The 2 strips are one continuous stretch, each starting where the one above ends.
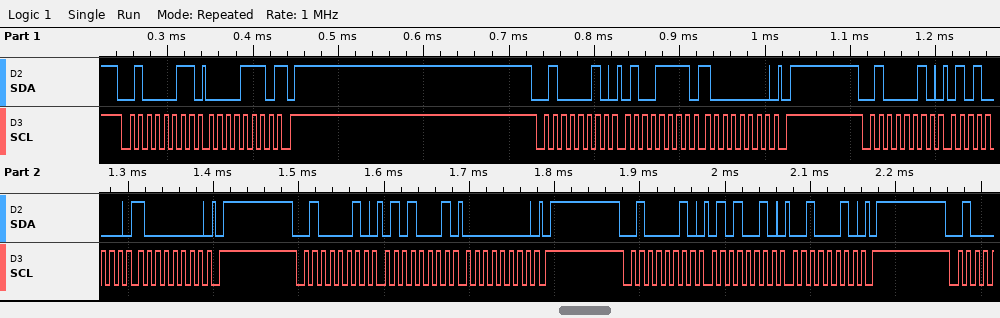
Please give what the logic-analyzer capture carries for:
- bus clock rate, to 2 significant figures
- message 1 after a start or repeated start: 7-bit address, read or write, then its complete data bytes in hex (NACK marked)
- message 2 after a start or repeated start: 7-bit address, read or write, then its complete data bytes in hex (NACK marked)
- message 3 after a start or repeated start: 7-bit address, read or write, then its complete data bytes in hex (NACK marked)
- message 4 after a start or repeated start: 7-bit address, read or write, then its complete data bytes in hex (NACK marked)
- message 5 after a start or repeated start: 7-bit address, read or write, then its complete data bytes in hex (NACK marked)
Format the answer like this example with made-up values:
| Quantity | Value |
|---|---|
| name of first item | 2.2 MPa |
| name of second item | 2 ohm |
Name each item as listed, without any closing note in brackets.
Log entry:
| Quantity | Value |
|---|---|
| bus clock rate, to 2 significant figures | 100 kHz |
| message 1 after a start or repeated start: 7-bit address, read or write, then its complete data bytes in hex | 0x21 read: 0E NACK |
| message 2 after a start or repeated start: 7-bit address, read or write, then its complete data bytes in hex | 0x21 write: 4F 80 |
| message 3 after a start or repeated start: 7-bit address, read or write, then its complete data bytes in hex | 0x21 write: 50 80 |
| message 4 after a start or repeated start: 7-bit address, read or write, then its complete data bytes in hex | 0x21 write: 51 00 |
| message 5 after a start or repeated start: 7-bit address, read or write, then its complete data bytes in hex | 0x21 write: 52 22 |
